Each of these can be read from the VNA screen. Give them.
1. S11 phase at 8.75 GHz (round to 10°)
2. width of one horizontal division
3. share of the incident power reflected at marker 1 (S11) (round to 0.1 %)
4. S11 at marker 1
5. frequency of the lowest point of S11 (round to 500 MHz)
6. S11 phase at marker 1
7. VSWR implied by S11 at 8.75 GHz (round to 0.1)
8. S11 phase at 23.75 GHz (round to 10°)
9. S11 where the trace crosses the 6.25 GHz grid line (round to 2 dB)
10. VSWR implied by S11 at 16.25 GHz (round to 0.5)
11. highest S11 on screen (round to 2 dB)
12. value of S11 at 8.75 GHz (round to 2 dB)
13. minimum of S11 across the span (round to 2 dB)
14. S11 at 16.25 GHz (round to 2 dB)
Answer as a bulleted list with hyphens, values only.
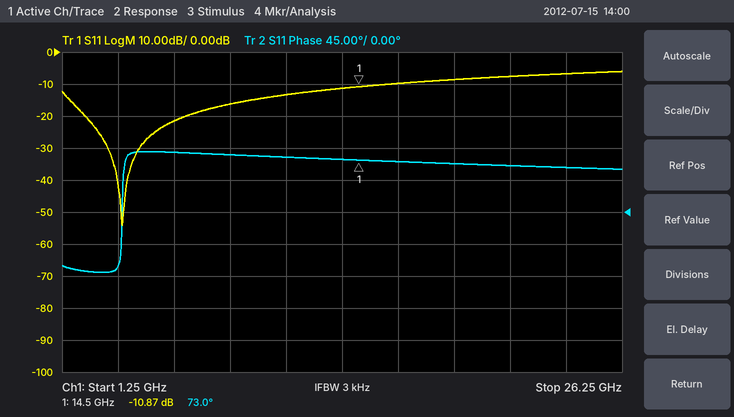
- 80°
- 2.5 GHz
- 8.2 %
- -10.87 dB
- 4.0 GHz
- 73.0°
- 1.4
- 60°
- -22 dB
- 2.0
- -6 dB
- -16 dB
- -54 dB
- -10 dB
